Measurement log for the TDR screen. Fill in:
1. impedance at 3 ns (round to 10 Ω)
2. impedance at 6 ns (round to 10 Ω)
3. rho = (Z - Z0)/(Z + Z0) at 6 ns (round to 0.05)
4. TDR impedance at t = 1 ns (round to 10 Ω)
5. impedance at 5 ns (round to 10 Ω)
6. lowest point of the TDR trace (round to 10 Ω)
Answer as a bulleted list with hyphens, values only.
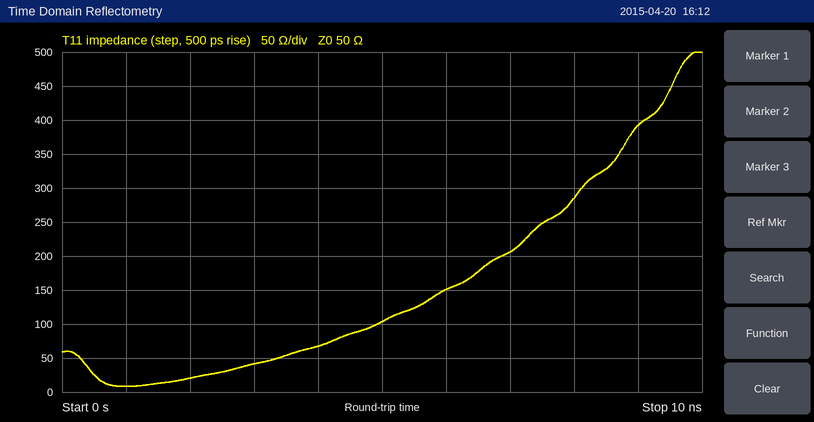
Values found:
- 40 Ω
- 150 Ω
- +0.50
- 10 Ω
- 100 Ω
- 10 Ω
